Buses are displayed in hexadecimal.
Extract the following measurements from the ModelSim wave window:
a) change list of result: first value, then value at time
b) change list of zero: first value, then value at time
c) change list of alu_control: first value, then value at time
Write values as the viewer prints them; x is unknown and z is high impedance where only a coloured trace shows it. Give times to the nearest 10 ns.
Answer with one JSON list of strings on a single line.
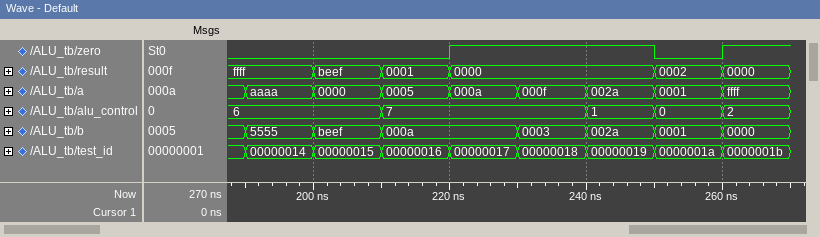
["ffff, beef at 200 ns, 0001 at 210 ns, 0000 at 220 ns, 0002 at 250 ns, 0000 at 260 ns", "0, 1 at 220 ns, 0 at 250 ns, 1 at 260 ns", "6, 7 at 210 ns, 1 at 240 ns, 0 at 250 ns, 2 at 260 ns"]
